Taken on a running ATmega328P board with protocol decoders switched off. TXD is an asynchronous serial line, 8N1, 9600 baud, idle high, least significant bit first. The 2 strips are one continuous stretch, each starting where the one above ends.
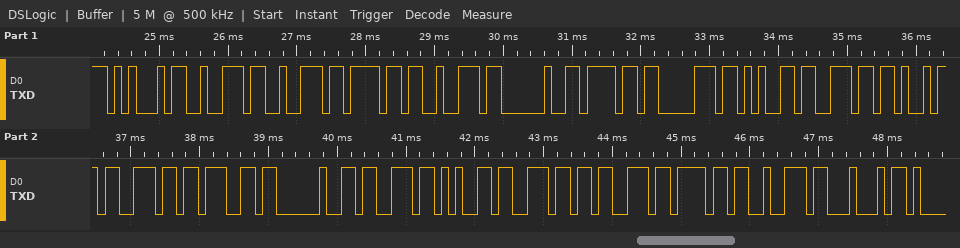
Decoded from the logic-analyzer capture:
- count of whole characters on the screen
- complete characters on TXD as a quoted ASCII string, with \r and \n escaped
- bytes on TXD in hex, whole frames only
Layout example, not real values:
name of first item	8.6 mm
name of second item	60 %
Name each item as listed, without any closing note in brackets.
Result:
count of whole characters on the screen	21
complete characters on TXD as a quoted ASCII string, with \r and \n escaped	"Error opening sensorD"
bytes on TXD in hex, whole frames only	45 72 72 6F 72 20 6F 70 65 6E 69 6E 67 20 73 65 6E 73 6F 72 44
